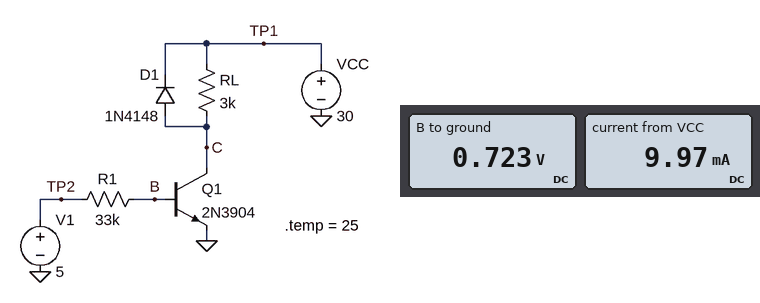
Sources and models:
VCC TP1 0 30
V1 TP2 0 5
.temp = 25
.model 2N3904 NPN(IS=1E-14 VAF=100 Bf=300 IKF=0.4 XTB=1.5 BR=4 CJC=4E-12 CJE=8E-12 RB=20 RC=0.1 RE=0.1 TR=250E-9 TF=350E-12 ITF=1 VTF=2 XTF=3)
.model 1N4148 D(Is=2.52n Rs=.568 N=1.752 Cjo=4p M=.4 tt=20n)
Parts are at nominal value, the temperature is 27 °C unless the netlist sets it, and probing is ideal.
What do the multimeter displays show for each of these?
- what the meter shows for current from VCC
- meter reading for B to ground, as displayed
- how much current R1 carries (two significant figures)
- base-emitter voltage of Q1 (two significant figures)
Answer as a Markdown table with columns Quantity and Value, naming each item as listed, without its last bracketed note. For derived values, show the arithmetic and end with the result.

| Quantity | Value |
|---|---|
| what the meter shows for current from VCC | 9.97 mA |
| meter reading for B to ground, as displayed | 0.723 V |
| how much current R1 carries | (5 V - 723 mV) / 33 kΩ = 130 µA |
| base-emitter voltage of Q1 | 723 mV = 720 mV |
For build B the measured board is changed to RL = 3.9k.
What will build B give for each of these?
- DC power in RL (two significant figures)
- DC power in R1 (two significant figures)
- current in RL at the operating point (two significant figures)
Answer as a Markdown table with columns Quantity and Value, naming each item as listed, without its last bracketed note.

| Quantity | Value |
|---|---|
| DC power in RL | 230 mW |
| DC power in R1 | 560 µW |
| current in RL at the operating point | 7.7 mA |
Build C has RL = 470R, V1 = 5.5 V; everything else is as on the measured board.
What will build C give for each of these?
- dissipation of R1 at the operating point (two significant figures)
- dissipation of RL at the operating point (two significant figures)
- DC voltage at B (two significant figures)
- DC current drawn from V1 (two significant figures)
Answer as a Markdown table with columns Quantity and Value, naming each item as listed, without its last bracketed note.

| Quantity | Value |
|---|---|
| dissipation of R1 at the operating point | 680 µW |
| dissipation of RL at the operating point | 850 mW |
| DC voltage at B | 760 mV |
| DC current drawn from V1 | 140 µA |
